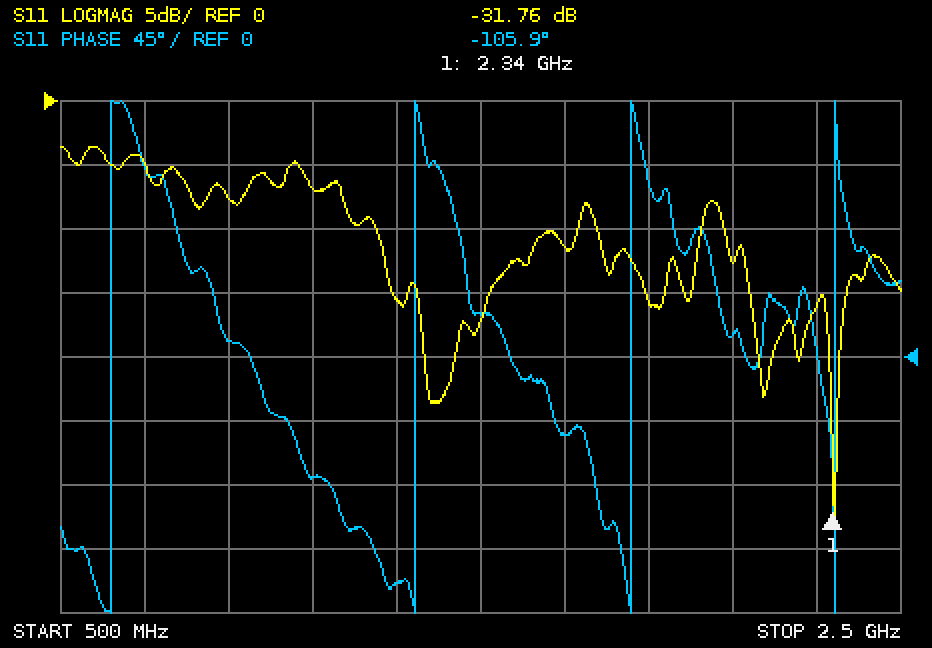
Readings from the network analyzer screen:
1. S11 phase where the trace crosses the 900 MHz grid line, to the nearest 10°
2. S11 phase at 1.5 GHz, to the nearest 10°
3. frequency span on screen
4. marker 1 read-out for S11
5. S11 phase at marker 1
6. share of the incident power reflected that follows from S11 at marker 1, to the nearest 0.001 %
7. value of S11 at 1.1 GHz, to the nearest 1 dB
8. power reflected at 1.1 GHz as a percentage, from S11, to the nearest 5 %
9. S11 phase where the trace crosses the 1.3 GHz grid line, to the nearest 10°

10°
30°
2 GHz
-31.76 dB
-105.9°
0.067 %
-7 dB
20 %
-160°
